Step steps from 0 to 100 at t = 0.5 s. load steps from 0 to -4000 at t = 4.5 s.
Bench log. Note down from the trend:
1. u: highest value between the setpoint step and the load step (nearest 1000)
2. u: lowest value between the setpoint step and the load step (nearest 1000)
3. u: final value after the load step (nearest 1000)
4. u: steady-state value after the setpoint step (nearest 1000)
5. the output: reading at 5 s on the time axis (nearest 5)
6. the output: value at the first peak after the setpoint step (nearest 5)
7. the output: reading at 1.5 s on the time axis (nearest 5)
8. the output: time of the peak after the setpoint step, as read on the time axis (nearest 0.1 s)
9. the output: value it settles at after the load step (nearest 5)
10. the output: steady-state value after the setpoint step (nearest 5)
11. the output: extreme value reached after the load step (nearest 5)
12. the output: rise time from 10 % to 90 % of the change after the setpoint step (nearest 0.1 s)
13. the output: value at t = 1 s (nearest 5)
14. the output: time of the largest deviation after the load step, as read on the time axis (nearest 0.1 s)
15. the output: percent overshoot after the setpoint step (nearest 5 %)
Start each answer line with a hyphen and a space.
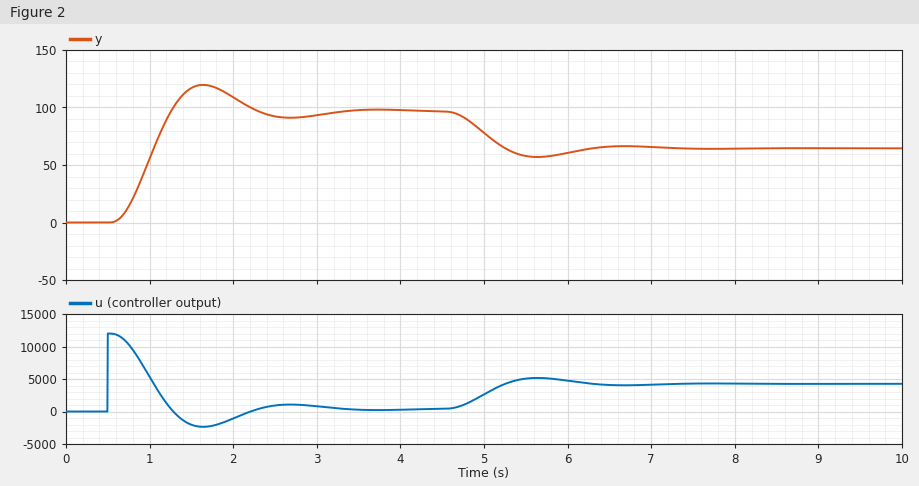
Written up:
- 12000
- -2000
- 4000
- 0
- 80
- 120
- 115
- 1.6 s
- 65
- 95
- 55
- 0.5 s
- 55
- 5.6 s
- 25 %
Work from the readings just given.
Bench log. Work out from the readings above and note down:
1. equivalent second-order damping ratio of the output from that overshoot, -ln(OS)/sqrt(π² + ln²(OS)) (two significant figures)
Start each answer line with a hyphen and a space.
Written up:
- 0.40
